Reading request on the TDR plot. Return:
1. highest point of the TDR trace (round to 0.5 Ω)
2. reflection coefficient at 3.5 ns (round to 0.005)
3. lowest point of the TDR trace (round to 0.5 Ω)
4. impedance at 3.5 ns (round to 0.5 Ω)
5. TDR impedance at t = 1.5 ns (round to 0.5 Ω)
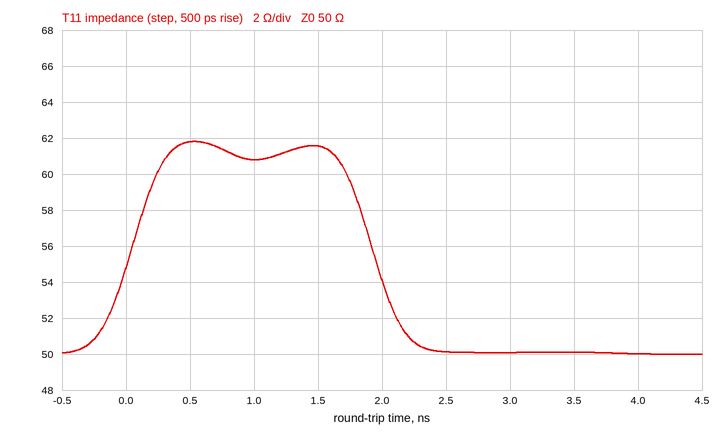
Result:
62.0 Ω
0.000
50.0 Ω
50.0 Ω
61.5 Ω
